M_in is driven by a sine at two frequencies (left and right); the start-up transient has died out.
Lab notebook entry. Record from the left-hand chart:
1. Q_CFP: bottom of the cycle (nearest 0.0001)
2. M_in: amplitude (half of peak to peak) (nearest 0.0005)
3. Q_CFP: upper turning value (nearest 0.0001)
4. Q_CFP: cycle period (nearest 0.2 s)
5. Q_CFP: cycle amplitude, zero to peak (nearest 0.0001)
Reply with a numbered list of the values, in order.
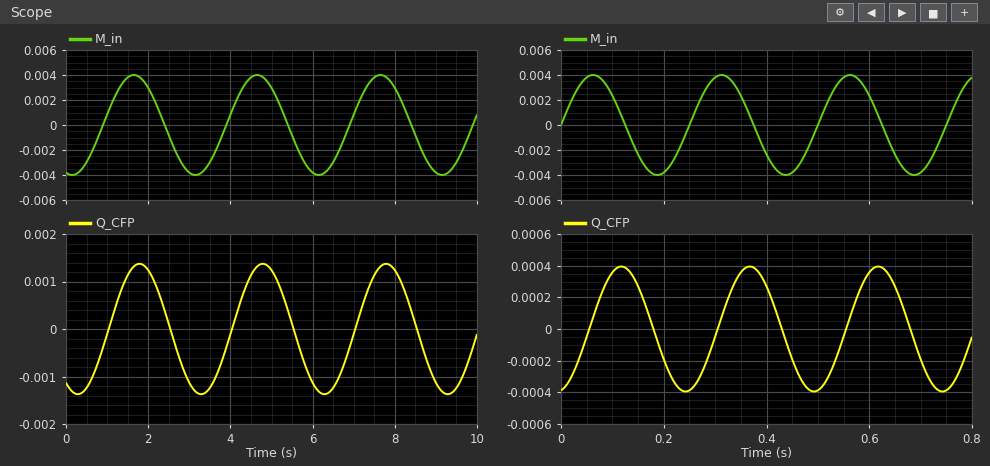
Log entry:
1. -0.0014
2. 0.0040
3. 0.0014
4. 3.0 s
5. 0.0014
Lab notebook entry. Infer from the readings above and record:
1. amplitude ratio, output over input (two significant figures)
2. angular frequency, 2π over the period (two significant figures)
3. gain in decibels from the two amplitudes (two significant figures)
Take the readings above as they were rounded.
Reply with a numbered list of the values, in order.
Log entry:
1. 0.35
2. 2.1 rad/s
3. -9.1 dB
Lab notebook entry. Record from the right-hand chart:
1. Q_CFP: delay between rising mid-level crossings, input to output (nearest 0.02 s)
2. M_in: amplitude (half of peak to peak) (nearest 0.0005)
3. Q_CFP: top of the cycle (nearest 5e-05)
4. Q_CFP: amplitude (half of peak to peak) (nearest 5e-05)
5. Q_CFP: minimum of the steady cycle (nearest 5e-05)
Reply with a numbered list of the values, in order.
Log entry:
1. 0.06 s
2. 0.0040
3. 0.00040
4. 0.00040
5. -0.00040
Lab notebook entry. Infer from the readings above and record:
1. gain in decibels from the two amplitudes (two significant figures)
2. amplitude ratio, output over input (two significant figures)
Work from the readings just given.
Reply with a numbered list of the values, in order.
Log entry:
1. -20 dB
2. 0.10
